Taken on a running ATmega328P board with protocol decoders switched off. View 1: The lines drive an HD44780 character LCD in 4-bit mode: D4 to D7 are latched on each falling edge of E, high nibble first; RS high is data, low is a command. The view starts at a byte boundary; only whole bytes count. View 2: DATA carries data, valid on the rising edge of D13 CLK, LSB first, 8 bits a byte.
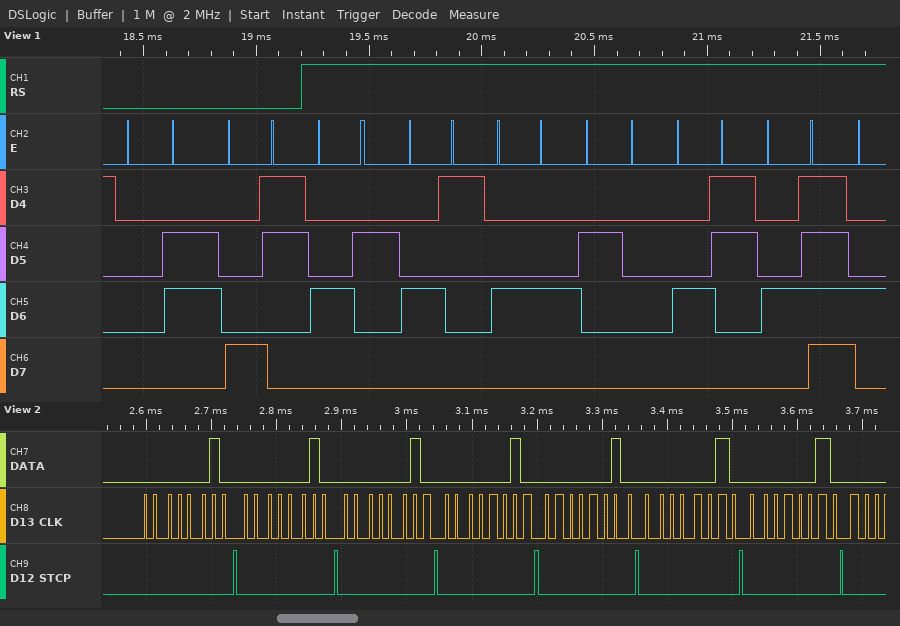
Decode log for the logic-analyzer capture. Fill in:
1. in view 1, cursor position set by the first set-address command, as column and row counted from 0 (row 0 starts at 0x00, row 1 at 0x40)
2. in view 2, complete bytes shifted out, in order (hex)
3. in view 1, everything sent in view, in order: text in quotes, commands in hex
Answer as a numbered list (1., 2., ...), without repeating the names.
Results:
1. column 3, row 0
2. 40 40 40 40 40 40 40
3. 0x06 0x83 "BAD CO"
